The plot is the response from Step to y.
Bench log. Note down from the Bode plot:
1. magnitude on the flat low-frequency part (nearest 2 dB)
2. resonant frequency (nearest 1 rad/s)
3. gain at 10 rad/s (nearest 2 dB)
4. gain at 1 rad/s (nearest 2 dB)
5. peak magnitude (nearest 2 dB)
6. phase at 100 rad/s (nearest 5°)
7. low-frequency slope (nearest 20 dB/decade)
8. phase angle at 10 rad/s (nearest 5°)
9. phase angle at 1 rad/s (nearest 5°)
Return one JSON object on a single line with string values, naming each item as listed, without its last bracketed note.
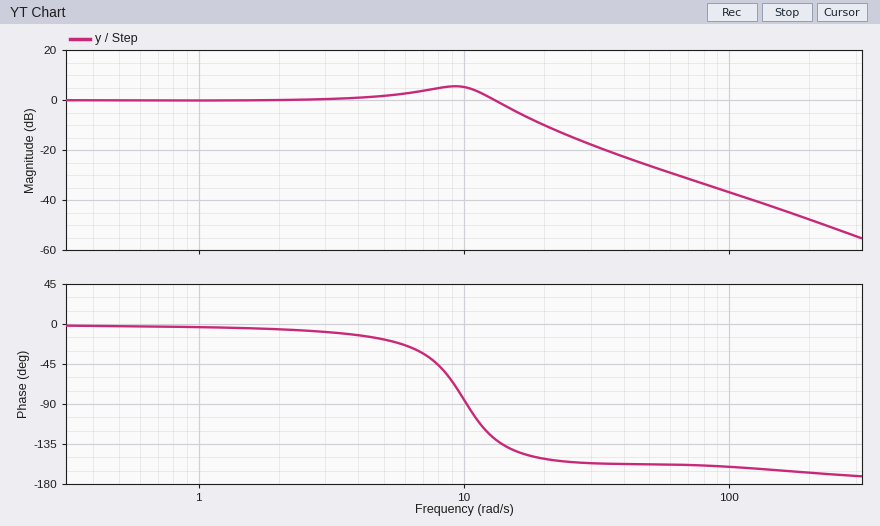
{"magnitude on the flat low-frequency part": "0 dB", "resonant frequency": "9 rad/s", "gain at 10 rad/s": "6 dB", "gain at 1 rad/s": "0 dB", "peak magnitude": "6 dB", "phase at 100 rad/s": "-160°", "low-frequency slope": "0 dB/decade", "phase angle at 10 rad/s": "-85°", "phase angle at 1 rad/s": "-5°"}
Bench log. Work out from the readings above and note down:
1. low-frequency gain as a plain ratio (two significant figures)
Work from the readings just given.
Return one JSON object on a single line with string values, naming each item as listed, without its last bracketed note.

{"low-frequency gain as a plain ratio": "1.0"}
